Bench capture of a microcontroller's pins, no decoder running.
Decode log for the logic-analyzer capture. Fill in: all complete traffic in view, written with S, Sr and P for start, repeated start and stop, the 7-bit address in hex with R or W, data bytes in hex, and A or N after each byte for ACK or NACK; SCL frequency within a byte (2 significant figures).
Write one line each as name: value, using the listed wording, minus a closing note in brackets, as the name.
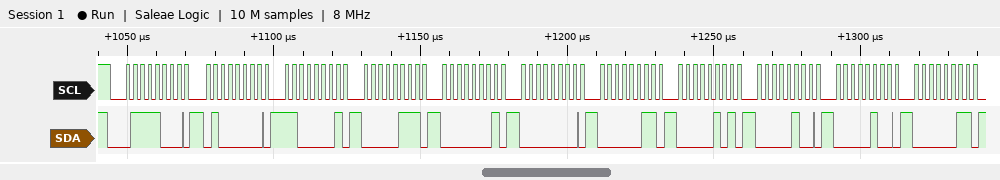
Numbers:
all complete traffic in view, written with S, Sr and P for start, repeated start and stop, the 7-bit address in hex with R or W, data bytes in hex, and A or N after each byte for ACK or NACK: S 3CW A 40 A C1 A 07 A 01 A 00 A 03 A 05 A 04 A 04 A 03 A
SCL frequency within a byte: 400 kHz
